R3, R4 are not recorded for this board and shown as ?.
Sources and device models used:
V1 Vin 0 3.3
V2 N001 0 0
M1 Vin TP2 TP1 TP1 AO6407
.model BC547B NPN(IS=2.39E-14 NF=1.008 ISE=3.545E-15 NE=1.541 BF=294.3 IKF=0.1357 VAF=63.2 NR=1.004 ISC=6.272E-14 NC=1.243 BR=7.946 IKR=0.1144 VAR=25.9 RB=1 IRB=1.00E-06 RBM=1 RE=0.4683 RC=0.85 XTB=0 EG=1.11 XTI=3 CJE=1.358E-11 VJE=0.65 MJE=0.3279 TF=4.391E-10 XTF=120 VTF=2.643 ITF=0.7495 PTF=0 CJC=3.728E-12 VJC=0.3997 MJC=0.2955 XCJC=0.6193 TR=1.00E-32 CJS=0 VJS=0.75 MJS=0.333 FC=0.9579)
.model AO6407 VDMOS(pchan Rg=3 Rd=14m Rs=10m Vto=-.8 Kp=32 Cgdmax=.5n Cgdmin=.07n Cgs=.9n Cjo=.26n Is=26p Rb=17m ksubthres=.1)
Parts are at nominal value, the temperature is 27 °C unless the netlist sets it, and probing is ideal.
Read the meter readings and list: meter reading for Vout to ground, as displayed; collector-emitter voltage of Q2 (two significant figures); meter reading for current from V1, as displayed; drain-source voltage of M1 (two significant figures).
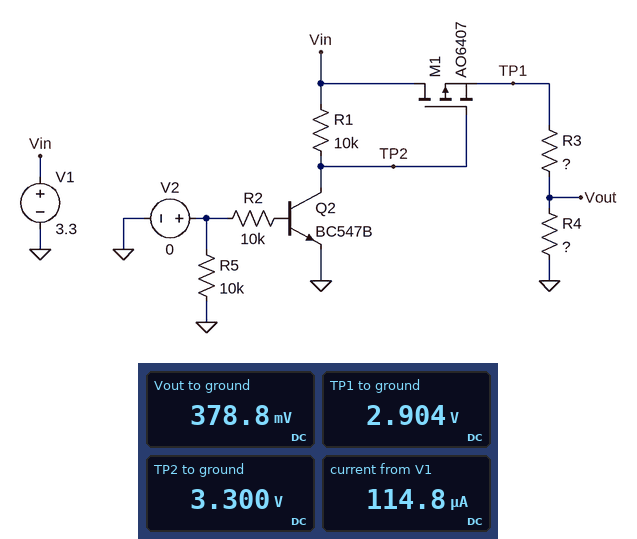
378.8 mV
3.3 V
114.8 µA
400 mV
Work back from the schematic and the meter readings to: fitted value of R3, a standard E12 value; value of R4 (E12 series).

22 kΩ
3.3 kΩ
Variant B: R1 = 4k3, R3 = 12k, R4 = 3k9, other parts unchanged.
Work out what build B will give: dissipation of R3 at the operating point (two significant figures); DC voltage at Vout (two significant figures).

400 µW
710 mV
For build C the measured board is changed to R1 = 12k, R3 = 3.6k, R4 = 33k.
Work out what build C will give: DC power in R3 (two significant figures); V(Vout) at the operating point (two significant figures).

23 µW
2.6 V
